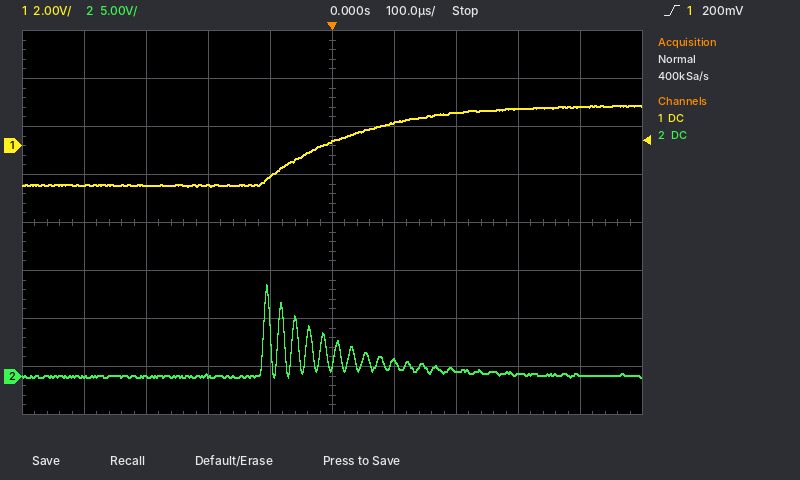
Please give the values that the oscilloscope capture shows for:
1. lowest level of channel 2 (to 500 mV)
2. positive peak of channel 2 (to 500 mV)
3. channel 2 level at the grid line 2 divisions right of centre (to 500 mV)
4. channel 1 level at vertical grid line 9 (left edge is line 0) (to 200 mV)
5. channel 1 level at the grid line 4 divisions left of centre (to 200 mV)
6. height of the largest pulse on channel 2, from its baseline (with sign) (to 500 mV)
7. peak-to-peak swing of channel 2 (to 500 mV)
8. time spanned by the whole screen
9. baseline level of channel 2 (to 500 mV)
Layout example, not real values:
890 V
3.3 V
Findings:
0.0 V
9.5 V
500 mV
1.6 V
-1.6 V
+9.5 V
9.5 V
1 ms
0.0 V
